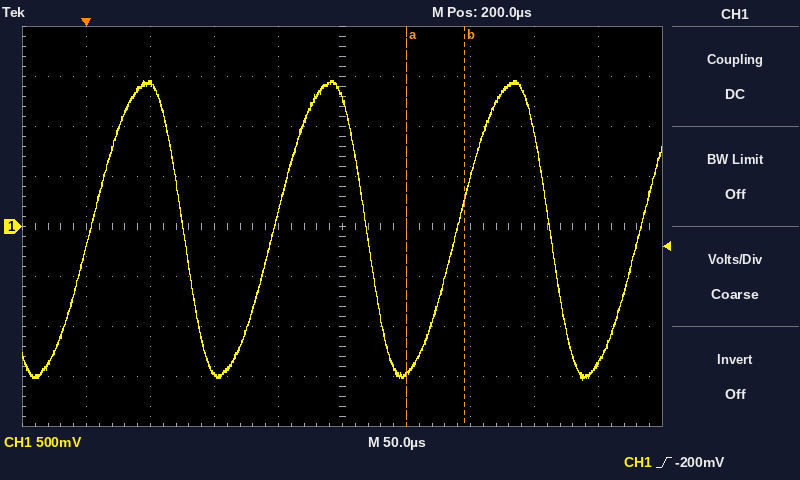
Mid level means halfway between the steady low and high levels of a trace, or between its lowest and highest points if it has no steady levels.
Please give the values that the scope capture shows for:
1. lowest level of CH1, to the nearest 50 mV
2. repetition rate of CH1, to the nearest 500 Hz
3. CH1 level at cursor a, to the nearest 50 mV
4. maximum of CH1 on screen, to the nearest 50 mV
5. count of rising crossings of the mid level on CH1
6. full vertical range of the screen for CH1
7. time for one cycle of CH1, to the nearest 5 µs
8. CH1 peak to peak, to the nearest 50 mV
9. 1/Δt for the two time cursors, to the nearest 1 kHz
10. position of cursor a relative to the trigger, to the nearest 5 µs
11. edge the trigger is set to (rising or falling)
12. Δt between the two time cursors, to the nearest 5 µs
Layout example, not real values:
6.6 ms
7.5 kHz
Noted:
-1.55 V
7.0 kHz
-1.45 V
1.45 V
4
4 V
145 µs
3.00 V
22 kHz
+250 µs
rising
45 µs
